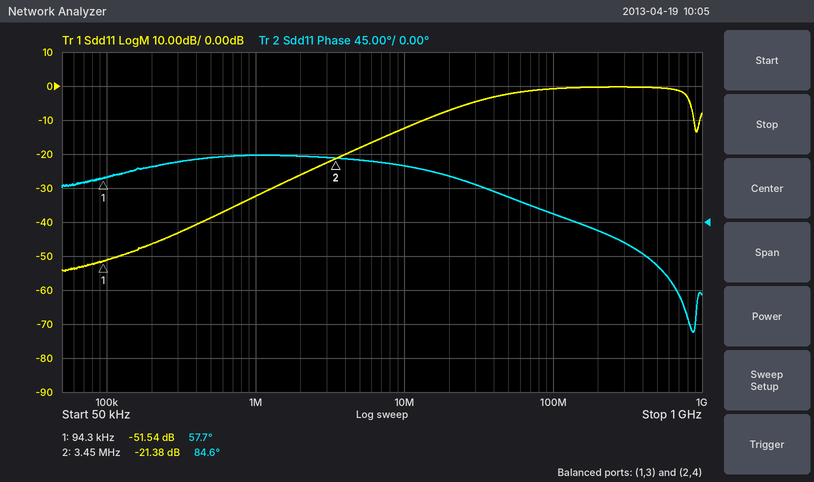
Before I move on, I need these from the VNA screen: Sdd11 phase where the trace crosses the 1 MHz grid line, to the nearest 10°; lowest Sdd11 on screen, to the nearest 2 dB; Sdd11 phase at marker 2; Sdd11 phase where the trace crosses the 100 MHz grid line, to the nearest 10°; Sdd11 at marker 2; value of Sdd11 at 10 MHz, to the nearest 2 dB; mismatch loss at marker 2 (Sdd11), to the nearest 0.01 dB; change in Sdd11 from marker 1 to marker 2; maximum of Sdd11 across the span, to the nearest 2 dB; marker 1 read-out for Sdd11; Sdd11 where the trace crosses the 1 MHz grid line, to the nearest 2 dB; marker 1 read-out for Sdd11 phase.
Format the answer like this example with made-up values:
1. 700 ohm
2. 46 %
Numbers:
1. 90°
2. -54 dB
3. 84.6°
4. 10°
5. -21.38 dB
6. -12 dB
7. 0.03 dB
8. 30.16 dB
9. 0 dB
10. -51.54 dB
11. -32 dB
12. 57.7°
